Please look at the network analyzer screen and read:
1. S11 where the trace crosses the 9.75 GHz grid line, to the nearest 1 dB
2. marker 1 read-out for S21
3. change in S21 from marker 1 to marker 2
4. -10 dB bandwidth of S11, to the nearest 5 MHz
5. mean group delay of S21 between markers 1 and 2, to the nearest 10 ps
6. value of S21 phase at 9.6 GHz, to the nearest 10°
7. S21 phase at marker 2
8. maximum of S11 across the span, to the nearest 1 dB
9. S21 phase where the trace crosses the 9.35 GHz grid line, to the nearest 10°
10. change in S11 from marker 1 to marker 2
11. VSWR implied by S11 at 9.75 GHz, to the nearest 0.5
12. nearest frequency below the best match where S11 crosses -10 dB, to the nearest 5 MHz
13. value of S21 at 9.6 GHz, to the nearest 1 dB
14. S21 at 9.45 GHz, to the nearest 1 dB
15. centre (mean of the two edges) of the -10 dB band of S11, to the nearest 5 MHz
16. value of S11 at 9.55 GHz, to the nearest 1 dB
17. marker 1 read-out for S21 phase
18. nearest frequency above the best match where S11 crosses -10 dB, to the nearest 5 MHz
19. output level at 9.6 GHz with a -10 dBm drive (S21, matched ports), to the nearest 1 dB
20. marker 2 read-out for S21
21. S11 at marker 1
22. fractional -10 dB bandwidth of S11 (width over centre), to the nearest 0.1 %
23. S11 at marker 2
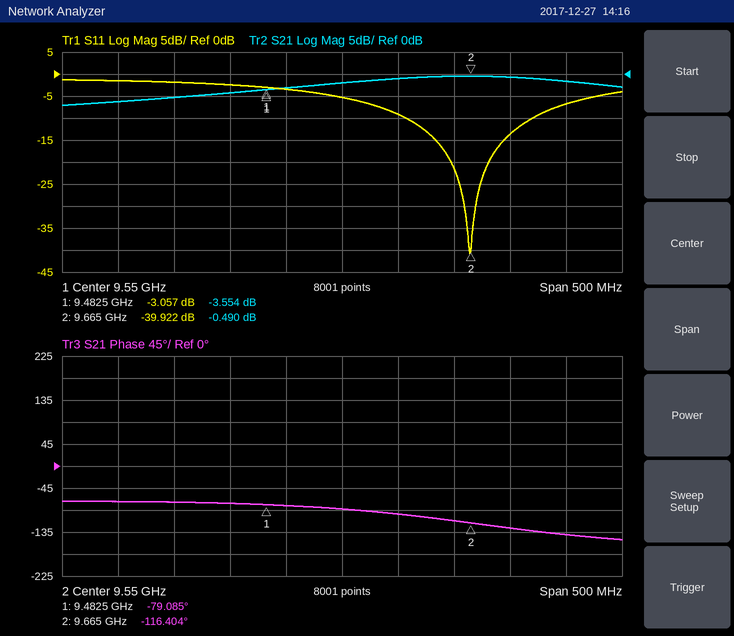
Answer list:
-7 dB
-3.554 dB
3.064 dB
115 MHz
570 ps
-100°
-116.404°
-1 dB
-70°
-36.865 dB
2.5
9.605 GHz
-1 dB
-4 dB
9.665 GHz
-5 dB
-79.085°
9.720 GHz
-11 dBm
-0.490 dB
-3.057 dB
1.2 %
-39.922 dB
